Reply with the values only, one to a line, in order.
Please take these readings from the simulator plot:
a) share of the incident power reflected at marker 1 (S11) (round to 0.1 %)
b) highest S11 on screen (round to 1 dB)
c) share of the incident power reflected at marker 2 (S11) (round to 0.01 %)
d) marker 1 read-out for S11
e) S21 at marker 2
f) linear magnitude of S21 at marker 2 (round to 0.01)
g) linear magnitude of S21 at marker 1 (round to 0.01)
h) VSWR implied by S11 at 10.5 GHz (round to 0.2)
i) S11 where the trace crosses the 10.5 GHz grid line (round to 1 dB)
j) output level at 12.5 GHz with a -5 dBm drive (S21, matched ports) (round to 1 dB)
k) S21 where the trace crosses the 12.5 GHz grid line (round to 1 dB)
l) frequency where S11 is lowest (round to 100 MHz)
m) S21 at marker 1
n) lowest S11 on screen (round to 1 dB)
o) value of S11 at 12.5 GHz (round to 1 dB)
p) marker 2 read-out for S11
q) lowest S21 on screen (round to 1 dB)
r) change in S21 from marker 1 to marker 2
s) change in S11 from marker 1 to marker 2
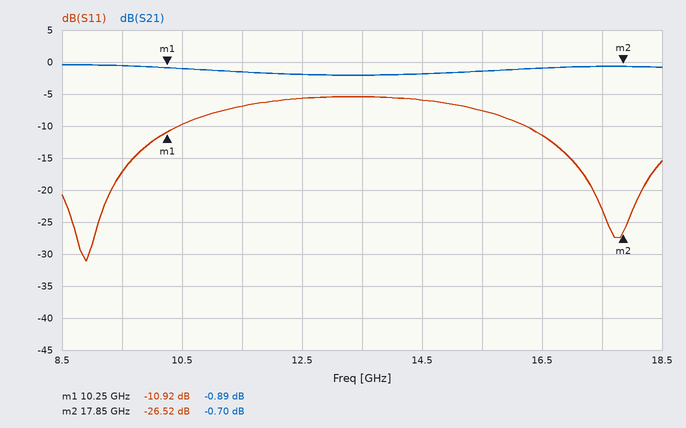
8.1 %
-5 dB
0.22 %
-10.92 dB
-0.70 dB
0.92
0.90
2.0
-10 dB
-7 dBm
-2 dB
8.9 GHz
-0.89 dB
-31 dB
-6 dB
-26.52 dB
-2 dB
0.19 dB
-15.60 dB
